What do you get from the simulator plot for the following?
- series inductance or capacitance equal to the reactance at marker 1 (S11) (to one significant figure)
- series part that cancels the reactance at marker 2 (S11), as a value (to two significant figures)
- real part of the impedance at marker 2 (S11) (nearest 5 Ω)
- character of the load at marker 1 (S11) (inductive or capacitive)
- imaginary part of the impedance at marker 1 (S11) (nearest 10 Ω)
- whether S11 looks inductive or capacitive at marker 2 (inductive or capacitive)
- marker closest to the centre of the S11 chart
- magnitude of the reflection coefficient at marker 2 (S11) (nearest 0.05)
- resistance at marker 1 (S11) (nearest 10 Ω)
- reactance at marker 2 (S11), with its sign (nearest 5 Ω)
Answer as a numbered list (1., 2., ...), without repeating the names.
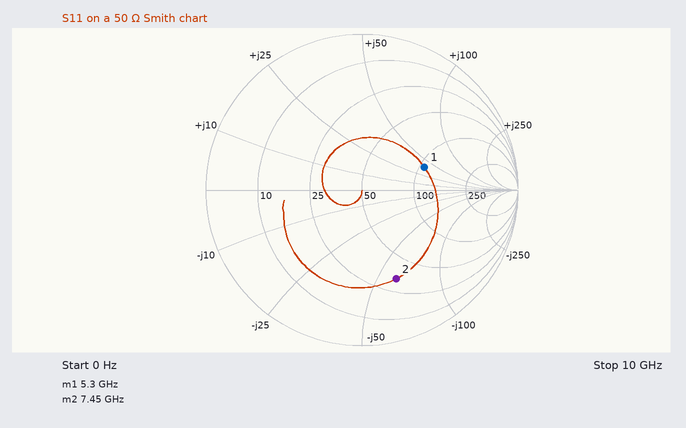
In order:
1. 1 nH
2. 1.3 nH
3. 35 Ω
4. inductive
5. +40 Ω
6. capacitive
7. marker 1
8. 0.60
9. 110 Ω
10. -60 Ω
